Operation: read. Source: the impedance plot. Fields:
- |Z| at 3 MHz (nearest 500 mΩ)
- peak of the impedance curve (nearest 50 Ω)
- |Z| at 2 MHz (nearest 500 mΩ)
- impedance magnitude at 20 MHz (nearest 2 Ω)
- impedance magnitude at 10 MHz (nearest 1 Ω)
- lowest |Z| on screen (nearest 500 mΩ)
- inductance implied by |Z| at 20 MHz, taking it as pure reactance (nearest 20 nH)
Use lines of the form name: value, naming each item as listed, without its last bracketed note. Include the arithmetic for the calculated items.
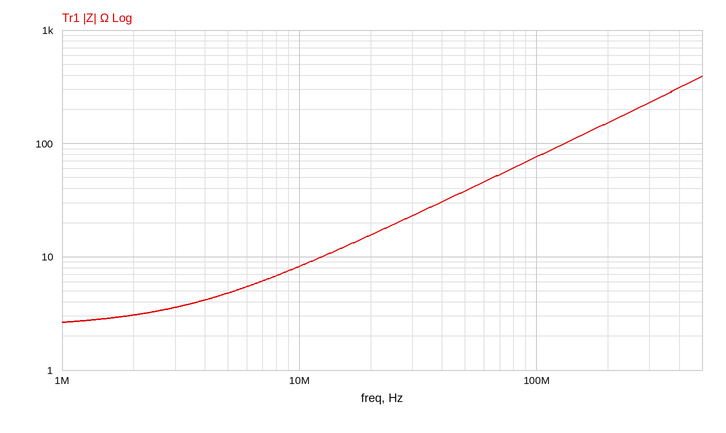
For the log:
|Z| at 3 MHz: 3.5 Ω
peak of the impedance curve: 400 Ω
|Z| at 2 MHz: 3.0 Ω
impedance magnitude at 20 MHz: 16 Ω
impedance magnitude at 10 MHz: 8 Ω
lowest |Z| on screen: 2.5 Ω
inductance implied by |Z| at 20 MHz, taking it as pure reactance: L = 16 Ω/(2π × 20 MHz) ≈ 127 nH, so 120 nH to the nearest 20 nH
